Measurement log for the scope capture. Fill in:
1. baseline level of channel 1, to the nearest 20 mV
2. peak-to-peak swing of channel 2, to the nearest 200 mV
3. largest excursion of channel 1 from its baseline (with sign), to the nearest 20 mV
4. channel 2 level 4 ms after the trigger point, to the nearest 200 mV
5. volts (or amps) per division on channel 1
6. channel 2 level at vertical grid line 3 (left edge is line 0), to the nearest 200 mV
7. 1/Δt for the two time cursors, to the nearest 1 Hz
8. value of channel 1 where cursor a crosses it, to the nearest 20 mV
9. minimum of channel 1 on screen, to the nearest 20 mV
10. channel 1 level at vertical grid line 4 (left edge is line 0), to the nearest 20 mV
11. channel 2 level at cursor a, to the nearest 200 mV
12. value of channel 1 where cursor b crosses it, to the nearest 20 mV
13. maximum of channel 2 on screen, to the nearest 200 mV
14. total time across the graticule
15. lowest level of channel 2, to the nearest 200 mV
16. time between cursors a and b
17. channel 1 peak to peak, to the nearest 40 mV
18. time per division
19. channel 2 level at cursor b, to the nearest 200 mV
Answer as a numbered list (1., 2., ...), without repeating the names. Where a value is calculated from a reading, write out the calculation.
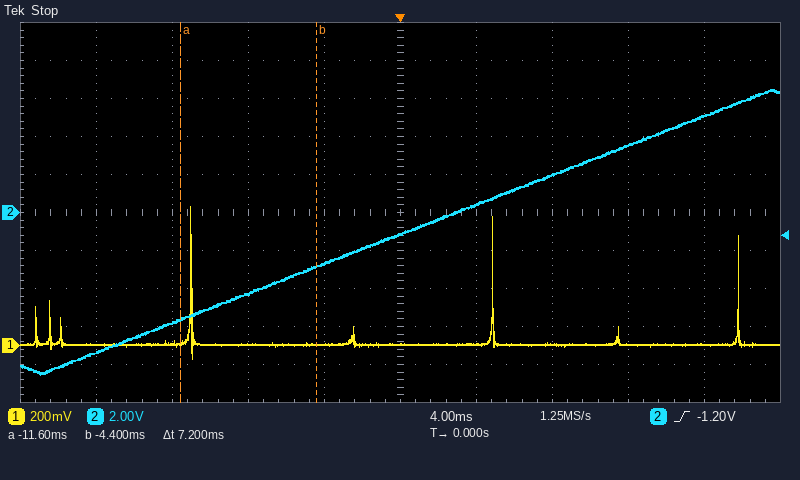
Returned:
1. 0 mV
2. 6.4 V − (-8.6 V) = 15.0 V
3. +720 mV
4. 400 mV
5. 200 mV
6. -4.2 V
7. 1 / 7.2 ms ≈ 139 Hz
8. 20 mV
9. -80 mV
10. 0 mV
11. -5.6 V
12. 0 mV
13. 6.4 V
14. 40 ms
15. -8.6 V
16. 7.2 ms
17. 800 mV
18. 4 ms
19. -2.8 V
